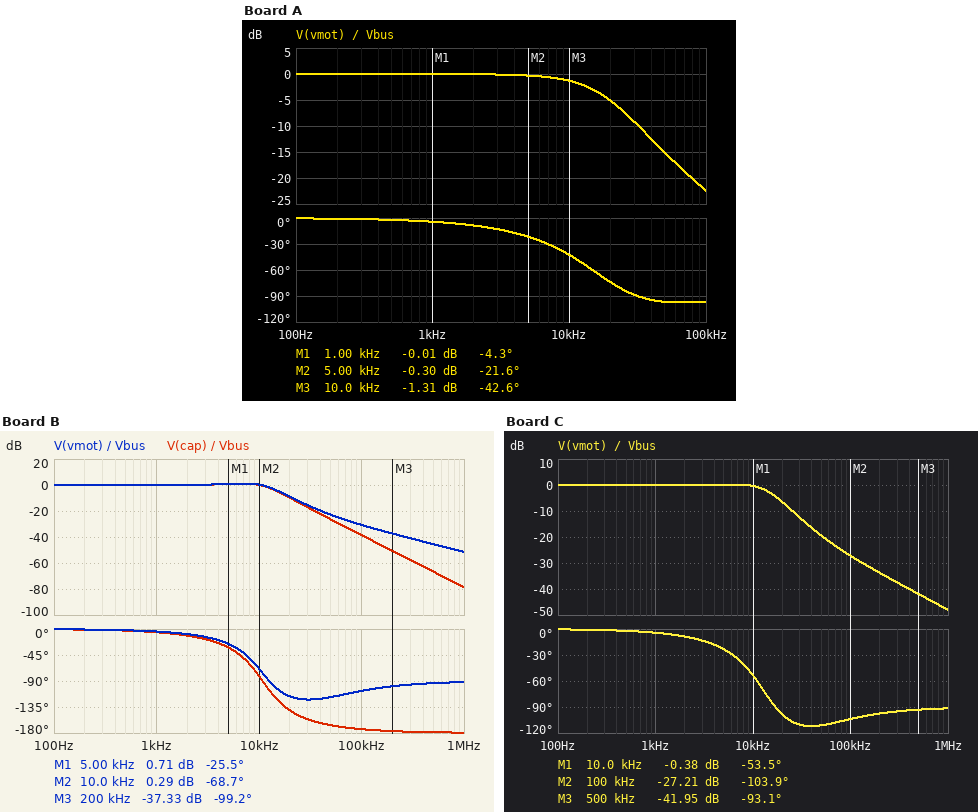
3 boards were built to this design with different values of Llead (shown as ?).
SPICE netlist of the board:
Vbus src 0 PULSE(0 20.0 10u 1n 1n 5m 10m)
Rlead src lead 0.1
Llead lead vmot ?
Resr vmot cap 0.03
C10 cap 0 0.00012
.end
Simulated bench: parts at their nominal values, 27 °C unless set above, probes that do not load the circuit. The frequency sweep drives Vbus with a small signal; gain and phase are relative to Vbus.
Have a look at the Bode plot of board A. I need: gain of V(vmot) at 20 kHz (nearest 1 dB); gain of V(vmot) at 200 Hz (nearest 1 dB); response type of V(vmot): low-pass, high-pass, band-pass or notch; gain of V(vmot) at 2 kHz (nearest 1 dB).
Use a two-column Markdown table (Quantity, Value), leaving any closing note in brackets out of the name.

| Quantity | Value |
|---|---|
| gain of V(vmot) at 20 kHz | -5 dB |
| gain of V(vmot) at 200 Hz | 0 dB |
| response type of V(vmot): low-pass, high-pass, band-pass or notch | low-pass |
| gain of V(vmot) at 2 kHz | 0 dB |
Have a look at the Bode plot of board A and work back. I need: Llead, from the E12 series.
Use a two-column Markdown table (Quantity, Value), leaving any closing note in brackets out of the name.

| Quantity | Value |
|---|---|
| Llead, from the E12 series | 680 nH |
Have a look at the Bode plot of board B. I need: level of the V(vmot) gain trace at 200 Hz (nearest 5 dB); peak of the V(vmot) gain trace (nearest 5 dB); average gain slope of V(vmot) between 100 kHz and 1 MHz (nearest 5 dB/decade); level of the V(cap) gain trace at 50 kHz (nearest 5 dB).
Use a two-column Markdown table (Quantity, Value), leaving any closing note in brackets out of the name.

| Quantity | Value |
|---|---|
| level of the V(vmot) gain trace at 200 Hz | 0 dB |
| peak of the V(vmot) gain trace | 0 dB |
| average gain slope of V(vmot) between 100 kHz and 1 MHz | -20 dB/decade |
| level of the V(cap) gain trace at 50 kHz | -25 dB |
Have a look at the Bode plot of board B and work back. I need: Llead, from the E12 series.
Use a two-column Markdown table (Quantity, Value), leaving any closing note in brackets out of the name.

| Quantity | Value |
|---|---|
| Llead, from the E12 series | 1.8 µH |
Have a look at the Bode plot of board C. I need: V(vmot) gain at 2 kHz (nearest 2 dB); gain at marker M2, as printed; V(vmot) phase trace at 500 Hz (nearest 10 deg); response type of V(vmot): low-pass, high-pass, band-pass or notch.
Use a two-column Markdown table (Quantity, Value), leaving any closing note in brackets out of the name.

| Quantity | Value |
|---|---|
| V(vmot) gain at 2 kHz | 0 dB |
| gain at marker M2, as printed | -27.21 dB |
| V(vmot) phase trace at 500 Hz | 0 deg |
| response type of V(vmot): low-pass, high-pass, band-pass or notch | low-pass |
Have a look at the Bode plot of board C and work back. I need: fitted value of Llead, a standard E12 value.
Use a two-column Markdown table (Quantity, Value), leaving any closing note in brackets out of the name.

| Quantity | Value |
|---|---|
| fitted value of Llead, a standard E12 value | 1.2 µH |
